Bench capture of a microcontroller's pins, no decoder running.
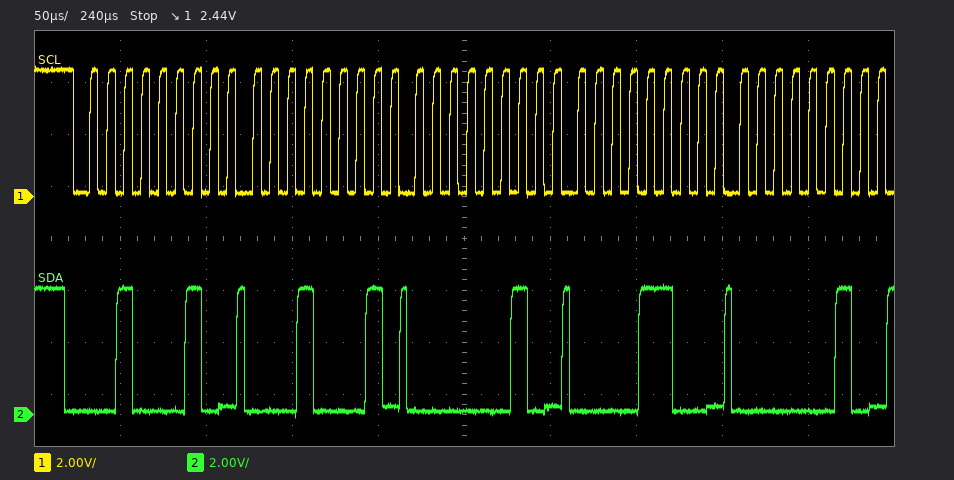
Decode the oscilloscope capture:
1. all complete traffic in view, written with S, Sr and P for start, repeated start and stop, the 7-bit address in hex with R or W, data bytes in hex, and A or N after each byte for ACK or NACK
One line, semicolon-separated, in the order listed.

S 11W A 11 A 02 A 0C A 02 A
